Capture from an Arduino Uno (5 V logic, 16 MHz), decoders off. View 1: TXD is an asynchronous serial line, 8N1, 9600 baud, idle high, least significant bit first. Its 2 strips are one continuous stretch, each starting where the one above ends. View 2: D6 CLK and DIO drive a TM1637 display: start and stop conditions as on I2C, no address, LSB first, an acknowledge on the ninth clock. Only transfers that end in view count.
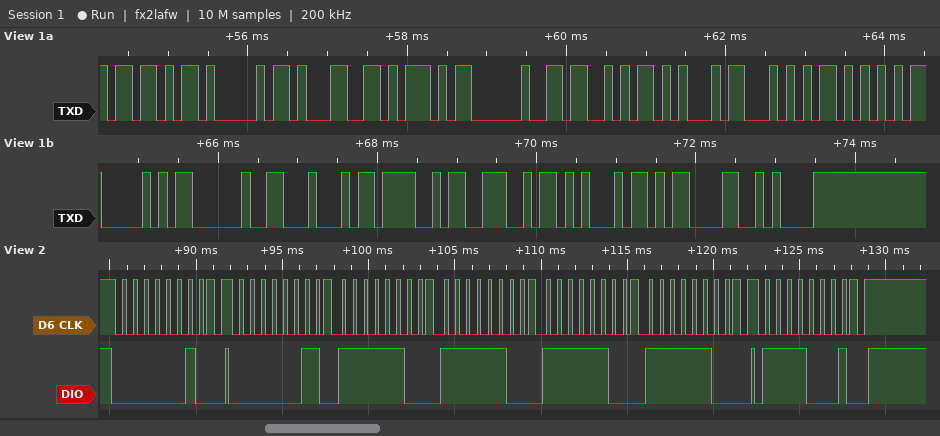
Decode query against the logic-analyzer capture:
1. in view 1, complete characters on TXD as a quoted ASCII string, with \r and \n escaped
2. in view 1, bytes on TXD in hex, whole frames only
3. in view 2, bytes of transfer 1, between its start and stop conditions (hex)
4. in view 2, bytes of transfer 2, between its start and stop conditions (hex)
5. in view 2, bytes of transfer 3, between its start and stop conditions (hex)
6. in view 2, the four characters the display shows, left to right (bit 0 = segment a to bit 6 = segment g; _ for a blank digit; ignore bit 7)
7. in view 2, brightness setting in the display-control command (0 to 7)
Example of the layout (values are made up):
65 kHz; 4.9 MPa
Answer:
"[A1] SETUP DONE\r\n"; 0x5B 0x41 0x31 0x5D 0x20 0x53 0x45 0x54 0x55 0x50 0x20 0x44 0x4F 0x4E 0x45 0x0D 0x0A; 40; C0 3F 3F 3F 3F; 8F; 0000; 7
